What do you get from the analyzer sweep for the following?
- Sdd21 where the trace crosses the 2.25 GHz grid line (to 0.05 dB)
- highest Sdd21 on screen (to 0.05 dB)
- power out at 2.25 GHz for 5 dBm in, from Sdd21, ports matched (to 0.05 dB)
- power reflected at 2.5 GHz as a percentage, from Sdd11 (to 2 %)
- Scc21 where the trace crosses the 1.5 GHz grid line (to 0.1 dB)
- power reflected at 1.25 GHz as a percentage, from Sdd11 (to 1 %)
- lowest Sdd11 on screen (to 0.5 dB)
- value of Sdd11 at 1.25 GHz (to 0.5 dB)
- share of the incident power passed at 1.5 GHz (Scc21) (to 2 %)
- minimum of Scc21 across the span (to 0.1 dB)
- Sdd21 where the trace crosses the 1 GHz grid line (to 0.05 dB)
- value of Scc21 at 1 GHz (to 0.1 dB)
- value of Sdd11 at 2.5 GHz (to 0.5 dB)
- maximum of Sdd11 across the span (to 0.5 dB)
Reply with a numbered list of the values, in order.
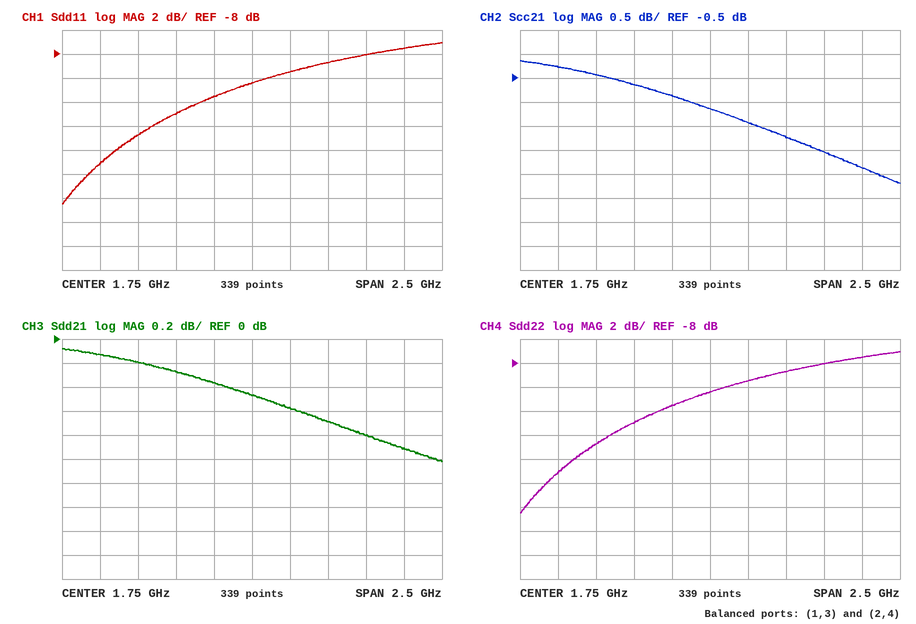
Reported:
1. -0.70 dB
2. -0.10 dB
3. 4.30 dBm
4. 16 %
5. -0.9 dB
6. 5 %
7. -20.5 dB
8. -13.0 dB
9. 82 %
10. -2.7 dB
11. -0.20 dB
12. -0.4 dB
13. -8.0 dB
14. -7.0 dB
